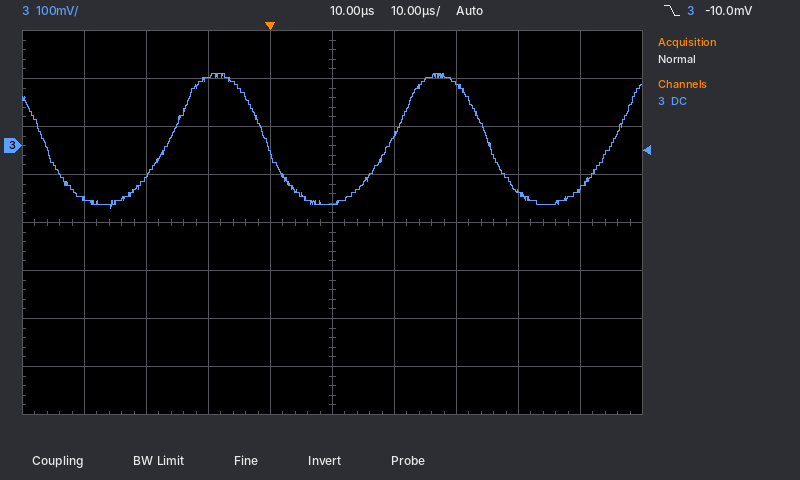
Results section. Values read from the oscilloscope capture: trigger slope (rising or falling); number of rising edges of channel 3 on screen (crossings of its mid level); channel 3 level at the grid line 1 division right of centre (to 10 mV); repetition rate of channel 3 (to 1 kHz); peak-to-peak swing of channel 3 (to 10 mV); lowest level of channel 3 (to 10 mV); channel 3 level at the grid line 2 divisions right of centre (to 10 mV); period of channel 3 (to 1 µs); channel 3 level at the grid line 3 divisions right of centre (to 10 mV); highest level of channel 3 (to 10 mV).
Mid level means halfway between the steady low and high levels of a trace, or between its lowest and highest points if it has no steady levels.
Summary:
falling
3
20 mV
28 kHz
280 mV
-130 mV
130 mV
36 µs
-100 mV
150 mV
